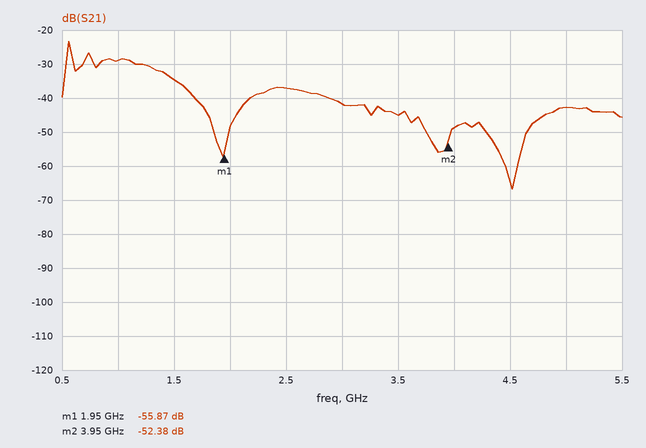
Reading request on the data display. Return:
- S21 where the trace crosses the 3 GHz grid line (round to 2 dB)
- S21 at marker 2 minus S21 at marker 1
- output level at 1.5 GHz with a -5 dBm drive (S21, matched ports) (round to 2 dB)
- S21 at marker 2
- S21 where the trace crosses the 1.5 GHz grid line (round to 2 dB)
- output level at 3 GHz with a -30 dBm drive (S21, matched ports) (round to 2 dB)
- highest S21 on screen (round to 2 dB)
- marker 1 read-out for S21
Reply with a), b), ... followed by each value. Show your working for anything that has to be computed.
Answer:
a) -42 dB
b) -52.38 − (-55.87) = 3.49 dB
c) -5 dBm + (-34 dB) = -40 dBm
d) -52.38 dB
e) -34 dB
f) -30 dBm + (-42 dB) = -72 dBm
g) -24 dB
h) -55.87 dB
